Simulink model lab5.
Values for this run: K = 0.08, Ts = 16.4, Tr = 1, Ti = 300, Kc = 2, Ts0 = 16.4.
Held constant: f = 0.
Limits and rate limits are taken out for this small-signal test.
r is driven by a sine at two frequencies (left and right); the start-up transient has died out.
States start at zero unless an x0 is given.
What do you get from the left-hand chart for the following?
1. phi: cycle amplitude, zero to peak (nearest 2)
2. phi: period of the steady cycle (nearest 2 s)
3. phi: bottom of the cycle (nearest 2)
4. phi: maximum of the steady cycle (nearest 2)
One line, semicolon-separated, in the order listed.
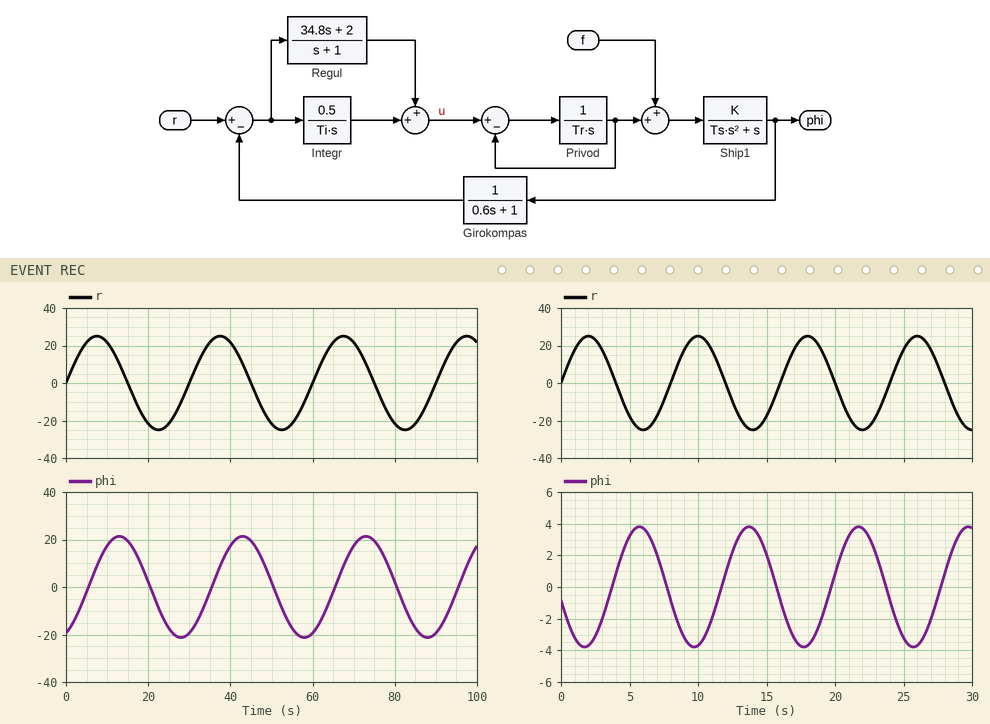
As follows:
22; 30 s; -22; 22
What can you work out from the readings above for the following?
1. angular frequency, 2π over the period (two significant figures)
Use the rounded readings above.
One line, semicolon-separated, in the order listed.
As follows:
0.21 rad/s
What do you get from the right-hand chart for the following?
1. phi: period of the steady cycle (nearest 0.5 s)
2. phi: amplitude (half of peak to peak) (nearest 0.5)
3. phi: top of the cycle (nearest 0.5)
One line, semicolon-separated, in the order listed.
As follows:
8.0 s; 4.0; 4.0
